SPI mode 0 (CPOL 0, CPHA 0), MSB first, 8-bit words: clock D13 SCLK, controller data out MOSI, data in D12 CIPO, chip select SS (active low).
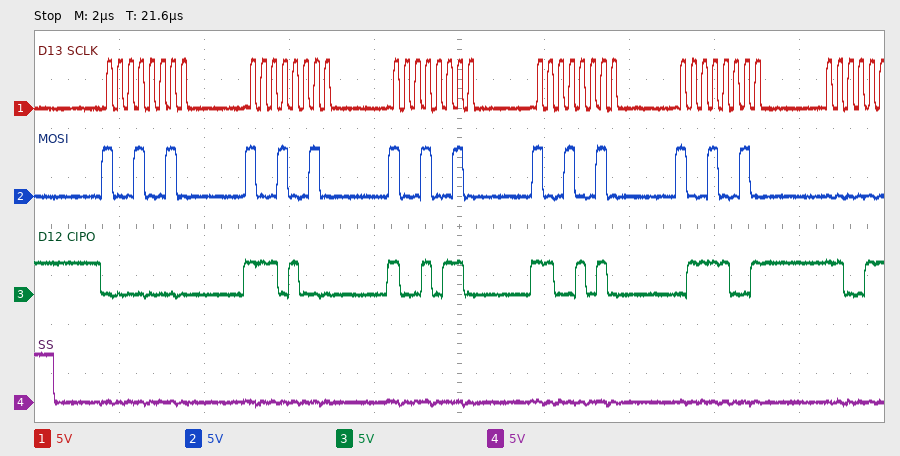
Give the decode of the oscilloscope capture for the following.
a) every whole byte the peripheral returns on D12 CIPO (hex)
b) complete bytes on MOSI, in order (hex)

00 E8 96 CA 79
92 92 92 92 92
